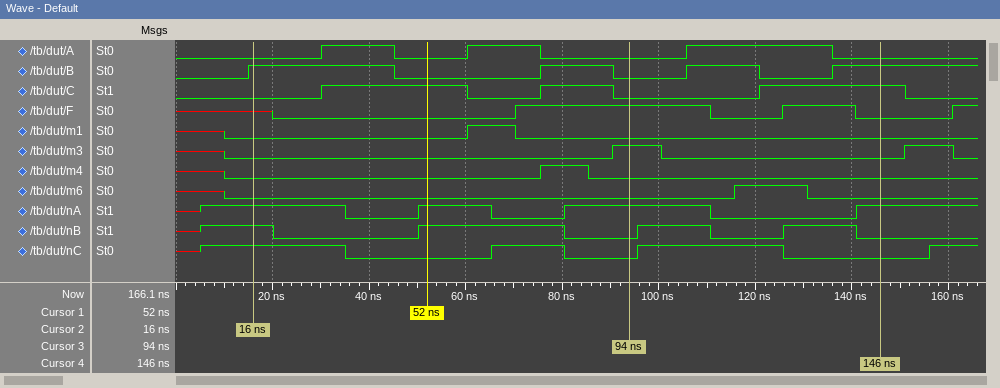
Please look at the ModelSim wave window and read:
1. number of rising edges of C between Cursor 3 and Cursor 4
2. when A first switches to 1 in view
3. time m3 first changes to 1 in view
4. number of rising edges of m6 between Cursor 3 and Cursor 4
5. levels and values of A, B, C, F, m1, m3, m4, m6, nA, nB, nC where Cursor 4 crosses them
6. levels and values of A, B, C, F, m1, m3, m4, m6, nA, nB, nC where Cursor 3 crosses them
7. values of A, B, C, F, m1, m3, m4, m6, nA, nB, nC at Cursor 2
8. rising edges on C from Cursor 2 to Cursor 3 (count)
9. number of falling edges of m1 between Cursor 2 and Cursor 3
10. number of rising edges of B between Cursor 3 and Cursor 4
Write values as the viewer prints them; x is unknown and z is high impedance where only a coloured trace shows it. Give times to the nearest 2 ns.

1
30 ns
90 ns
1
A=0, B=1, C=1, F=0, m1=0, m3=0, m4=0, m6=0, nA=1, nB=0, nC=0
A=0, B=0, C=0, F=1, m1=0, m3=1, m4=0, m6=0, nA=1, nB=0, nC=0
A=0, B=1, C=0, F=x, m1=0, m3=0, m4=0, m6=0, nA=1, nB=1, nC=1
2
1
2
